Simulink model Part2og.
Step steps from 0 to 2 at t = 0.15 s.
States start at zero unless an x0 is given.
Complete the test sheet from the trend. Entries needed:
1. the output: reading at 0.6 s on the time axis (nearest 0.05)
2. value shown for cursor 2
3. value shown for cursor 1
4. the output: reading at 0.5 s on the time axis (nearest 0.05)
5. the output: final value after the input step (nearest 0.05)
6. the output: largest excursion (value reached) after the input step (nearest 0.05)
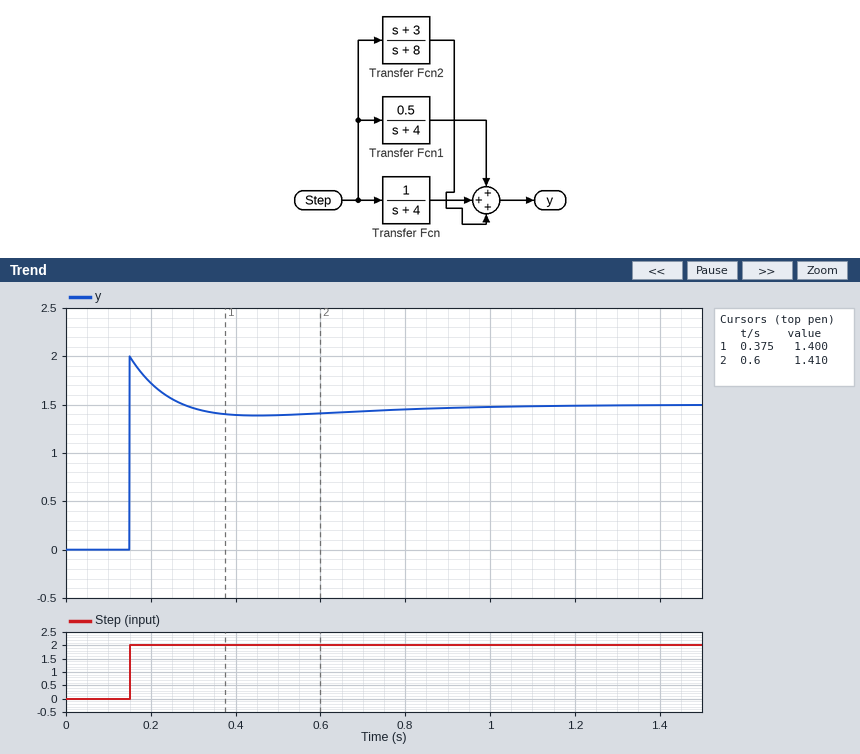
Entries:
1.40
1.410
1.400
1.40
1.50
2.00
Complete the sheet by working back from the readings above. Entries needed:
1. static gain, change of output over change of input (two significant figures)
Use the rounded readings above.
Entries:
0.75
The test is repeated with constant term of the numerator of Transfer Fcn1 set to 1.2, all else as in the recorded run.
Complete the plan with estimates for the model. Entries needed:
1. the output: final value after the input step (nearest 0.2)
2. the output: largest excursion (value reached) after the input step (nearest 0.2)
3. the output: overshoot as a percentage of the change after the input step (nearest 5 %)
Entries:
1.8
2.0
10 %
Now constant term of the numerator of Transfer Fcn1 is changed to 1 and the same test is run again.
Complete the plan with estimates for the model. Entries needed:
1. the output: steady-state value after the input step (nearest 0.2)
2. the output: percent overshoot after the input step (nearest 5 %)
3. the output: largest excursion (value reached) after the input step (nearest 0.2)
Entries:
1.8
15 %
2.0
